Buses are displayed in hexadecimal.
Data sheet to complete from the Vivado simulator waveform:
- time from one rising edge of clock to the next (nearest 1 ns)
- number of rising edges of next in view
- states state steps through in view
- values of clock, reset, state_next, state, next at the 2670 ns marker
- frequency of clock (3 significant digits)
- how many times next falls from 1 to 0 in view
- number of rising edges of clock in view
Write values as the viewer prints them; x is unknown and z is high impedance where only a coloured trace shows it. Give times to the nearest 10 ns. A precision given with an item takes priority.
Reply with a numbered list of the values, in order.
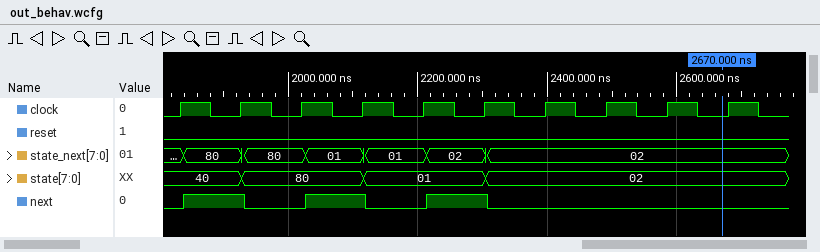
1. 94 ns
2. 3
3. 40, 80, 01, 02
4. clock=0, reset=0, state_next=02, state=02, next=0
5. 10.6 MHz
6. 3
7. 10
